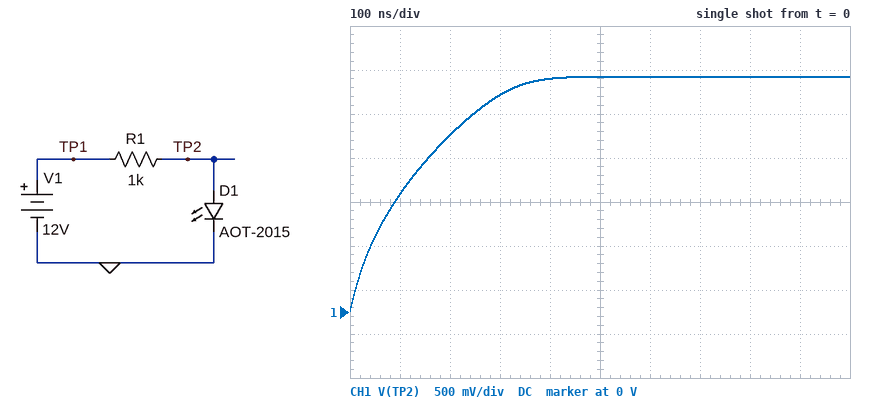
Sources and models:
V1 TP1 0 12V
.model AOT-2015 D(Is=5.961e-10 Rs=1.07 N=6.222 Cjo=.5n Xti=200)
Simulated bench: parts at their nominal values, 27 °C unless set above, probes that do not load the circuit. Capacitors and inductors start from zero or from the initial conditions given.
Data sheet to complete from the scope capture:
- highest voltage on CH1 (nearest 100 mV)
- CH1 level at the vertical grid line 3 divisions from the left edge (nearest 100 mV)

2.7 V
2.5 V
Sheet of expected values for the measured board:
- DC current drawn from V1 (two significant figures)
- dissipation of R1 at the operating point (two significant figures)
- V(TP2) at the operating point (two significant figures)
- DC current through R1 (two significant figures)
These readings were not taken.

9.3 mA
87 mW
2.7 V
9.3 mA
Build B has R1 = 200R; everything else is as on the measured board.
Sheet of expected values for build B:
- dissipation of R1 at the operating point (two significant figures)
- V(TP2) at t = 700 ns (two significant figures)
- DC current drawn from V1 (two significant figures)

410 mW
3.0 V
45 mA
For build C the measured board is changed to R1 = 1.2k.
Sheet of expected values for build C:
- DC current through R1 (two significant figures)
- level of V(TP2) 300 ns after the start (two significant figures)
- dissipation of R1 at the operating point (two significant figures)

7.8 mA
2.3 V
73 mW
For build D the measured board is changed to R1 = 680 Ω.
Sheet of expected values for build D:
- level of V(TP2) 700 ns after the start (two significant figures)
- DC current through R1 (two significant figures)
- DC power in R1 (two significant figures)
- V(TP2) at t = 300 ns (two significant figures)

2.7 V
14 mA
130 mW
2.7 V
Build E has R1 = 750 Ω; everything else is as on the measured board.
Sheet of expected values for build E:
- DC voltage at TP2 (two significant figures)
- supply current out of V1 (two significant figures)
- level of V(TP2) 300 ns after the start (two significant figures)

2.7 V
12 mA
2.7 V
